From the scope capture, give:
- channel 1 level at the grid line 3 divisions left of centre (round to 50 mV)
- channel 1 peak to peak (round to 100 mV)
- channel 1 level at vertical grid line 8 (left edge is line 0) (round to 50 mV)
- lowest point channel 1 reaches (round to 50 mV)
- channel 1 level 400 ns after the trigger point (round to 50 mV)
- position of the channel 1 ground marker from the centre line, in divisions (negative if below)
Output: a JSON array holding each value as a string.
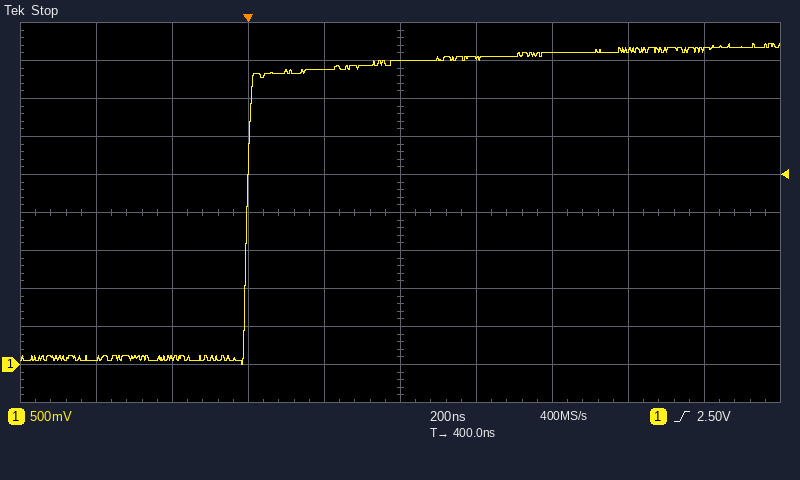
["100 mV", "4.20 V", "4.15 V", "0 mV", "4.00 V", "-4.0 div"]
